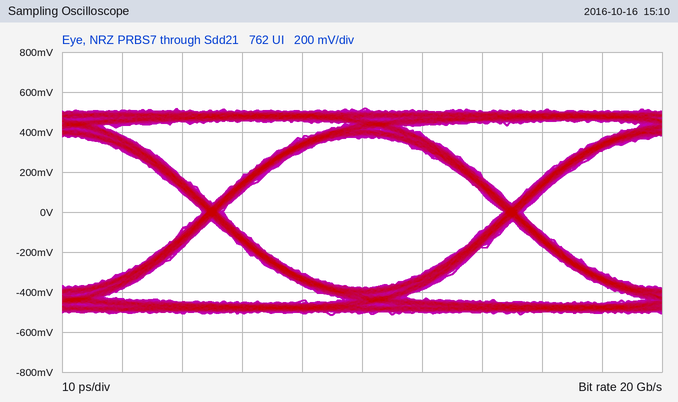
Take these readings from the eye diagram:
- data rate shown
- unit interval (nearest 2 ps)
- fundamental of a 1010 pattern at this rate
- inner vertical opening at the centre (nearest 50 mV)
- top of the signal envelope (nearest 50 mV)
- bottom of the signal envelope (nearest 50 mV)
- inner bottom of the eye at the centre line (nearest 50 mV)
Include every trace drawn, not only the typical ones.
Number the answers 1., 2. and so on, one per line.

1. 20 Gb/s
2. 50 ps
3. 10 GHz
4. 750 mV
5. 500 mV
6. -500 mV
7. -400 mV
